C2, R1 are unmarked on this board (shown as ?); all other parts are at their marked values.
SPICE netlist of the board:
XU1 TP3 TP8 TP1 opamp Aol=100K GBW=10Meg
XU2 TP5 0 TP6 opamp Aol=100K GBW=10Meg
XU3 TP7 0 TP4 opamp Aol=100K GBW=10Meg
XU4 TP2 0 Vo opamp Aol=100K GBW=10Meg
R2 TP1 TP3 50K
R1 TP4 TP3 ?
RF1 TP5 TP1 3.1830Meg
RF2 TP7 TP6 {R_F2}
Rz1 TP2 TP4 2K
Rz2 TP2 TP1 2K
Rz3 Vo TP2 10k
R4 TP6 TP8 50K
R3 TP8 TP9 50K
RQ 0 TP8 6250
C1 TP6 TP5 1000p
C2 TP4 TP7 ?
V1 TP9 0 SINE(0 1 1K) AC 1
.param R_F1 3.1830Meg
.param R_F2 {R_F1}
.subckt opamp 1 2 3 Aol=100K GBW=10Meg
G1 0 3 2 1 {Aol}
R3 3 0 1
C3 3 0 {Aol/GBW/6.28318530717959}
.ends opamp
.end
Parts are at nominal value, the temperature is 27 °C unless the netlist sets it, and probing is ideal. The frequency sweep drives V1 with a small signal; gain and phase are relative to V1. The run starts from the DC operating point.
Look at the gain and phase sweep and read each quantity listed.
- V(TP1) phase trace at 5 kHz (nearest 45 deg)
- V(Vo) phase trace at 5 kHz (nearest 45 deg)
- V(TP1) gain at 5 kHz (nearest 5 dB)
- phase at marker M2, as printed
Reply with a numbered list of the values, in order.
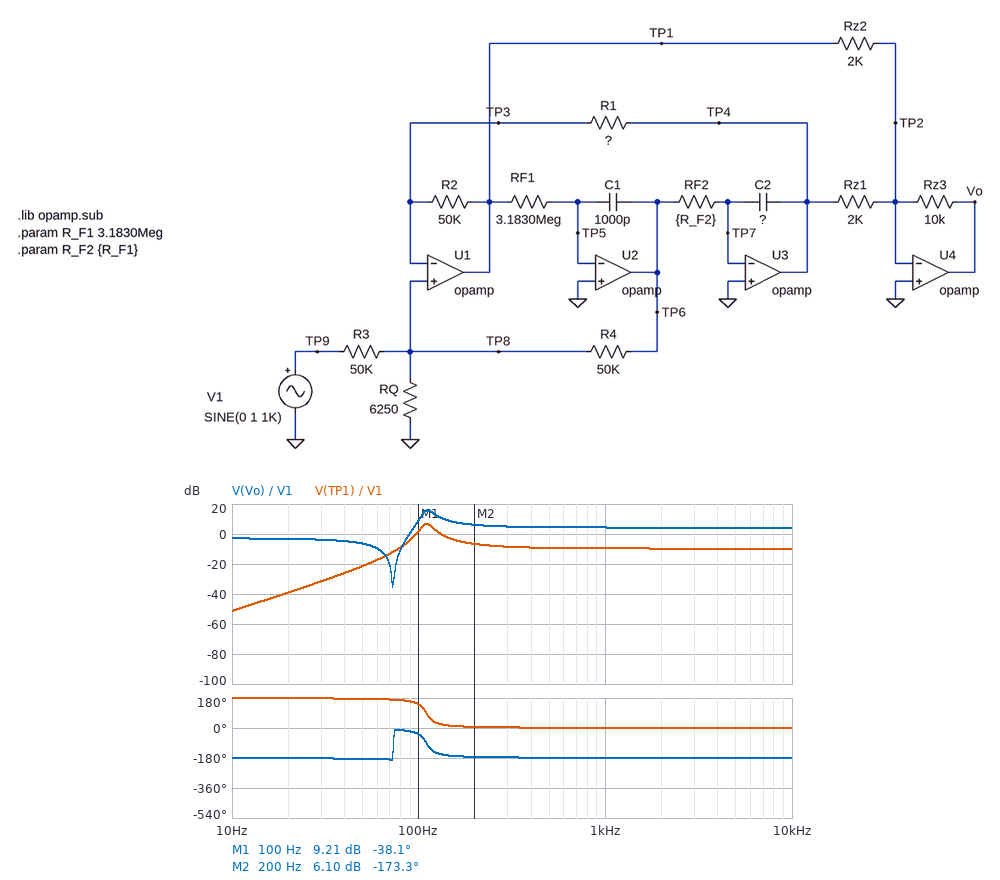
1. 0 deg
2. -180 deg
3. -10 dB
4. -173.3 deg
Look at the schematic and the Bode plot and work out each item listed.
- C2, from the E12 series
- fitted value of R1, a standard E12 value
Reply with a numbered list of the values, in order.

1. 470 pF
2. 22 kΩ
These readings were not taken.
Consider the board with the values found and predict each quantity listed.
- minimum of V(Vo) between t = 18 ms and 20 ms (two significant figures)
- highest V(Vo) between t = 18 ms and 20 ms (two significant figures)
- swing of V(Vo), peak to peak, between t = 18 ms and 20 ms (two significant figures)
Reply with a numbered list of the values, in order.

1. -1.6 V
2. 1.7 V
3. 3.3 V
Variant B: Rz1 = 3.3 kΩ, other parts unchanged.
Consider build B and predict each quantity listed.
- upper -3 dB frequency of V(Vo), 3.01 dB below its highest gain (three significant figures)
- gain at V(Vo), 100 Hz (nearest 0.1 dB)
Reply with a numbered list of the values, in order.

1. 121 Hz
2. 12.4 dB
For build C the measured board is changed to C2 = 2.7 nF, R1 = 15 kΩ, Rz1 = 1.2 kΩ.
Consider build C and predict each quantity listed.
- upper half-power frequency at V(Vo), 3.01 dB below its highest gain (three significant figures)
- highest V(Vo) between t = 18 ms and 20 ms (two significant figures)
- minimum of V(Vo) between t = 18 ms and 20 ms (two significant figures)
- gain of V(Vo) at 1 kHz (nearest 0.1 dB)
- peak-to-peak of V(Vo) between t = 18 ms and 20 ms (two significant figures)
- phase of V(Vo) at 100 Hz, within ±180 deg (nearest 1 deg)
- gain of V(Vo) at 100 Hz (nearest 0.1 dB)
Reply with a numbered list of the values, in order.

1. 161 Hz
2. 2.2 V
3. -2.2 V
4. 6.7 dB
5. 4.3 V
6. -163 deg
7. 8.1 dB
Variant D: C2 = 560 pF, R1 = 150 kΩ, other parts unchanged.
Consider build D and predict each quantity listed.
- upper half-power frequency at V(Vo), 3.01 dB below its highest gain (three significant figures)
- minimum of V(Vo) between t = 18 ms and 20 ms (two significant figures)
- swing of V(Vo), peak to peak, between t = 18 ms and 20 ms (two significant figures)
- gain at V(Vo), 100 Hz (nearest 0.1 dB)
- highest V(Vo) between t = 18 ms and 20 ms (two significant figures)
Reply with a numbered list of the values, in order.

1. 41.0 Hz
2. -630 mV
3. 1.3 V
4. -7.3 dB
5. 700 mV
